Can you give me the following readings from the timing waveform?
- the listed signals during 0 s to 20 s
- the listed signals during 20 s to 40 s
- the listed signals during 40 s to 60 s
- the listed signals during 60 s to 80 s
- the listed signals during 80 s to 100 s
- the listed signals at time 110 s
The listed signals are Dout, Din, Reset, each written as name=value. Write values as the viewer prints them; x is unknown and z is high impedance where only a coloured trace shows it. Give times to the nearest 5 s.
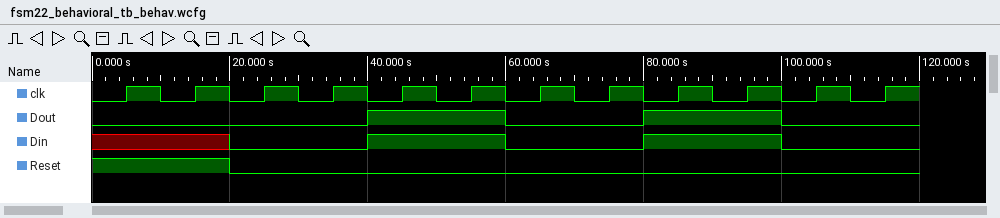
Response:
Dout=0, Din=x, Reset=1
Dout=0, Din=0, Reset=0
Dout=1, Din=1, Reset=0
Dout=0, Din=0, Reset=0
Dout=1, Din=1, Reset=0
Dout=0, Din=0, Reset=0
